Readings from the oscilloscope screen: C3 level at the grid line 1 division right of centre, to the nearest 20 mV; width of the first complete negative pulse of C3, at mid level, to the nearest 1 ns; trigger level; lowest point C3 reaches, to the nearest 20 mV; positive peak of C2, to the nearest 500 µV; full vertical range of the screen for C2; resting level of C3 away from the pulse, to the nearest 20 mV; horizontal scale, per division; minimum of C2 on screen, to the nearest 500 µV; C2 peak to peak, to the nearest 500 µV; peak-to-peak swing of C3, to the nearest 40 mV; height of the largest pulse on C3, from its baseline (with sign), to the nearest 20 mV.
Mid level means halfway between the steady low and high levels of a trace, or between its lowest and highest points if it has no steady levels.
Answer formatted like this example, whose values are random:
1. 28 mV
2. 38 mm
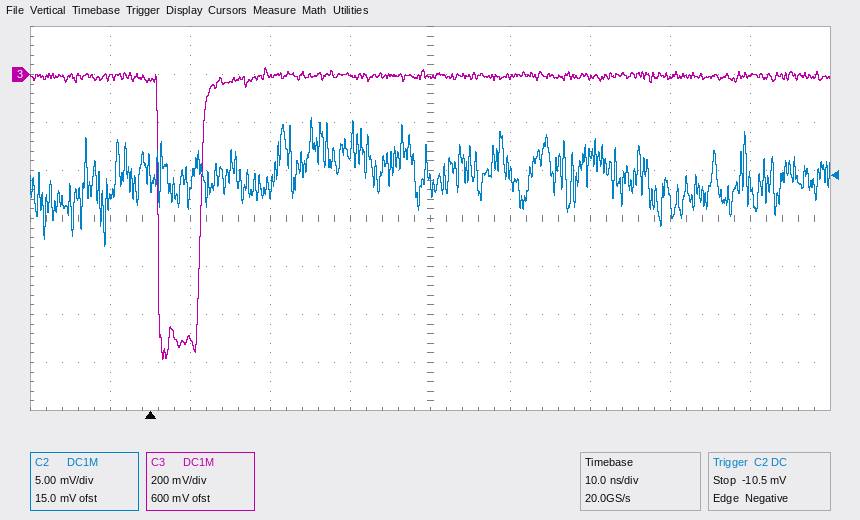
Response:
1. 0 mV
2. 5 ns
3. -10.5 mV
4. -1.18 V
5. -4.5 mV
6. 40 mV
7. 0 mV
8. 10 ns
9. -18.0 mV
10. 13.5 mV
11. 1.20 V
12. -1.18 V
